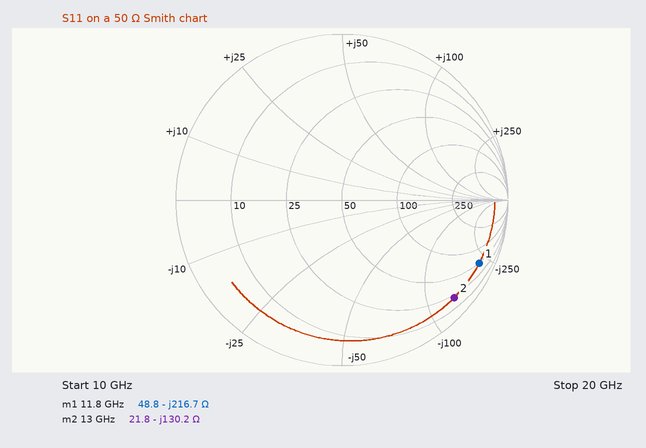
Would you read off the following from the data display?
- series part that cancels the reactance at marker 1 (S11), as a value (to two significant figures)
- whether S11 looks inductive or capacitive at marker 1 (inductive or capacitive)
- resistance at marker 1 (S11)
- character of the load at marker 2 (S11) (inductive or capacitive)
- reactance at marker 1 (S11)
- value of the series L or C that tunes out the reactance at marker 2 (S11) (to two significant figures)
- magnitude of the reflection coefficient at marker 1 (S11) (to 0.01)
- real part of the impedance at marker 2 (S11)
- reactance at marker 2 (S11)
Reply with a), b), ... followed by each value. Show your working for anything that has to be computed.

a) L = 216.7 Ω/(2π × 11.8 GHz) ≈ 2.9 nH
b) capacitive
c) 48.8 Ω
d) capacitive
e) -216.7 Ω
f) L = 130.2 Ω/(2π × 13 GHz) ≈ 1.6 nH
g) 0.91
h) 21.8 Ω
i) -130.2 Ω
